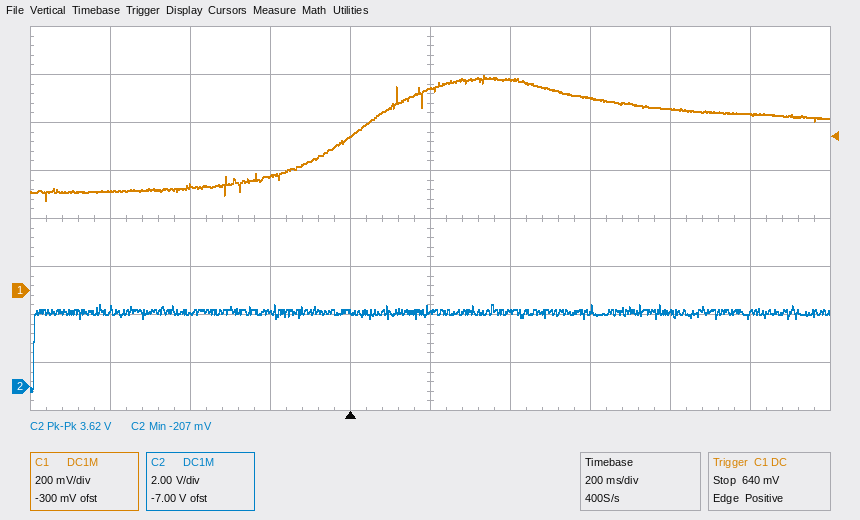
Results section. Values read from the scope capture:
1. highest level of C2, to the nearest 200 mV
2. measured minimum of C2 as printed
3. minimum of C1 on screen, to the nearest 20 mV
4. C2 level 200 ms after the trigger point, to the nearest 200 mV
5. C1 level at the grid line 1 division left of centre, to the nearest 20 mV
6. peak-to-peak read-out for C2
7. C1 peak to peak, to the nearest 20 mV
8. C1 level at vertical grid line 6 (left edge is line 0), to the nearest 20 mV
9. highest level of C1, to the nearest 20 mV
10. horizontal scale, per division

3.4 V
-207 mV
380 mV
3.2 V
640 mV
3.62 V
520 mV
880 mV
900 mV
200 ms
